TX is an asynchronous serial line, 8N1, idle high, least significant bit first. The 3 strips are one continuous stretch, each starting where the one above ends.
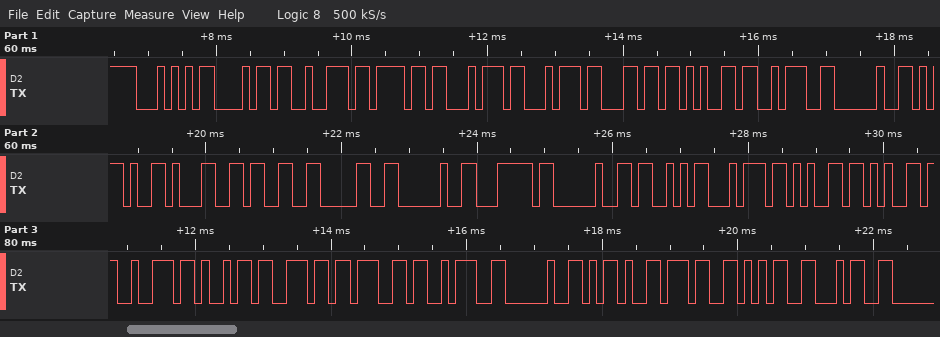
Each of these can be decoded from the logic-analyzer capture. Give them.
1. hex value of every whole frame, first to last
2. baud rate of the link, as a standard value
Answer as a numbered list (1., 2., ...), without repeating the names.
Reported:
1. 54 68 72 6F 74 74 6C 65 3A 20 2D 31 33 30 20 7C 20 53 74 65 65 72 69 6E 67 3A 20 2D 37 35 34
2. 9600 baud
